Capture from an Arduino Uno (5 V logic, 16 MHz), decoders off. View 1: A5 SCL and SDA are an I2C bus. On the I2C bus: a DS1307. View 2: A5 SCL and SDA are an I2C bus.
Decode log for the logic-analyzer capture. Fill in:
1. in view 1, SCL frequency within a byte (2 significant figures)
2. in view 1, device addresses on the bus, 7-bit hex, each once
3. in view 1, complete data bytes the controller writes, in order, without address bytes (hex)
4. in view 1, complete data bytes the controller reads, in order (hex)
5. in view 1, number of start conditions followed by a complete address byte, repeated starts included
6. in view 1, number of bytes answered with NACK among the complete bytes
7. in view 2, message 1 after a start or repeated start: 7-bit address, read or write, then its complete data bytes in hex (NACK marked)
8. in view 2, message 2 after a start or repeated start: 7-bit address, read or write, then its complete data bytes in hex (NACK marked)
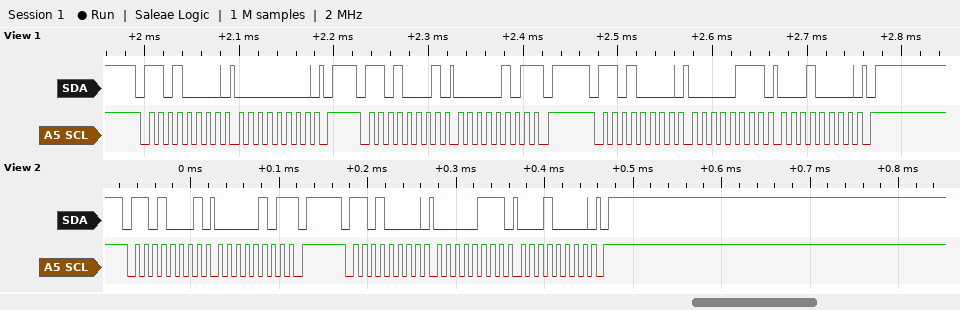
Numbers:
100 kHz
0x68
00 07 10
05
3
1
0x68 read: 05 NACK
0x68 write: 07 10
